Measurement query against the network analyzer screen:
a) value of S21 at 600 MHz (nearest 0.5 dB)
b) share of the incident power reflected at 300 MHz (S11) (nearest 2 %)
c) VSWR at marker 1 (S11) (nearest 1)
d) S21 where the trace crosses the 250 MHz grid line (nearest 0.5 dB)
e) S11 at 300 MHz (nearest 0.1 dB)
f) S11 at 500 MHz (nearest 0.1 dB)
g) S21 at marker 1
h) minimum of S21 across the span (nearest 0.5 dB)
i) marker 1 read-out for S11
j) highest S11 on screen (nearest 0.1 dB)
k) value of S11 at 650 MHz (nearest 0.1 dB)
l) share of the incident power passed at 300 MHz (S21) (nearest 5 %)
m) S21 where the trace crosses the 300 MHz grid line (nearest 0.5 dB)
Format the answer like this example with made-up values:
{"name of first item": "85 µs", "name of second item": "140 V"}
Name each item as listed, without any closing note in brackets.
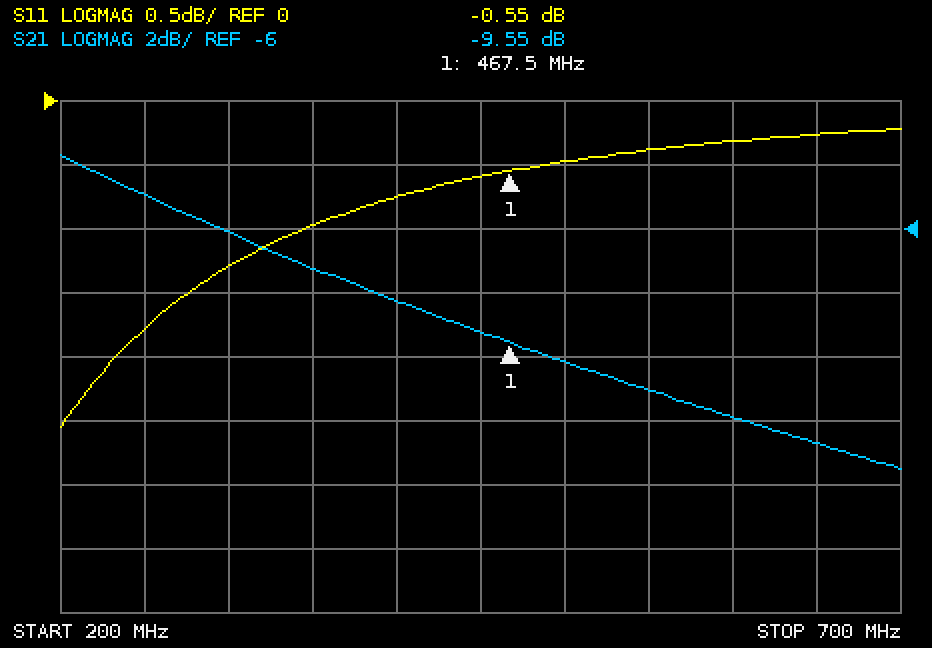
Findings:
{"value of S21 at 600 MHz": "-12.0 dB", "share of the incident power reflected at 300 MHz (S11)": "74 %", "VSWR at marker 1 (S11)": "32", "S21 where the trace crosses the 250 MHz grid line": "-5.0 dB", "S11 at 300 MHz": "-1.3 dB", "S11 at 500 MHz": "-0.5 dB", "S21 at marker 1": "-9.55 dB", "minimum of S21 across the span": "-13.5 dB", "marker 1 read-out for S11": "-0.55 dB", "highest S11 on screen": "-0.2 dB", "value of S11 at 650 MHz": "-0.3 dB", "share of the incident power passed at 300 MHz (S21)": "25 %", "S21 where the trace crosses the 300 MHz grid line": "-6.0 dB"}
